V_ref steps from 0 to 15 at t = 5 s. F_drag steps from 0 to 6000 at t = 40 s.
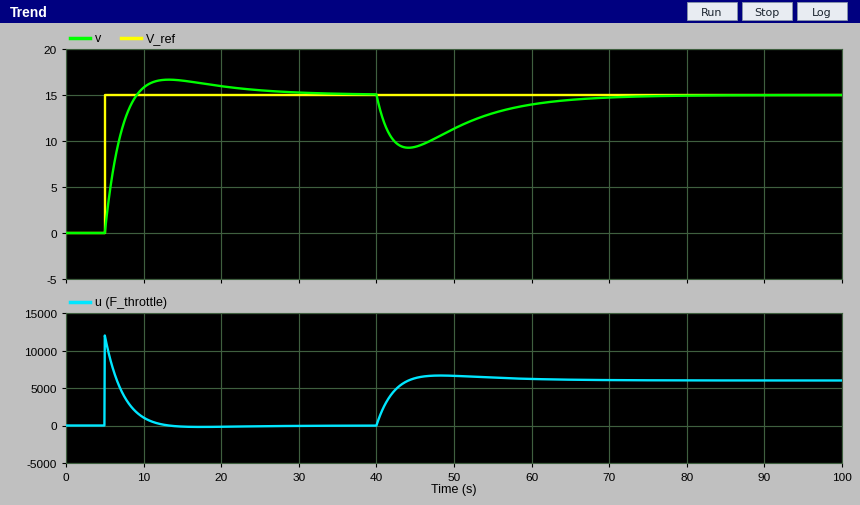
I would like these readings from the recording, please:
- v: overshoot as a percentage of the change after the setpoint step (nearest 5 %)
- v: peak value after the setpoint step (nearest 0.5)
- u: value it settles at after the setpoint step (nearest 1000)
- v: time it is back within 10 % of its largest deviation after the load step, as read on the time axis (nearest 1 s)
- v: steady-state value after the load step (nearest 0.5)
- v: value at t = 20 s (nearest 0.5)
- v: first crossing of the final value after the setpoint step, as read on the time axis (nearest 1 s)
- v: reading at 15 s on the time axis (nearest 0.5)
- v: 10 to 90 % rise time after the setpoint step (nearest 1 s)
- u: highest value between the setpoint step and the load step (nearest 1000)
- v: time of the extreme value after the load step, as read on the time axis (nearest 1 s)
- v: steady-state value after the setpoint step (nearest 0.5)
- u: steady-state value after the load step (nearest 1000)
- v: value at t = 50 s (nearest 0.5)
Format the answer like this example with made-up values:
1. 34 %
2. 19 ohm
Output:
1. 10 %
2. 16.5
3. 0
4. 64 s
5. 15.0
6. 16.0
7. 9 s
8. 16.5
9. 3 s
10. 12000
11. 44 s
12. 15.0
13. 6000
14. 11.5
